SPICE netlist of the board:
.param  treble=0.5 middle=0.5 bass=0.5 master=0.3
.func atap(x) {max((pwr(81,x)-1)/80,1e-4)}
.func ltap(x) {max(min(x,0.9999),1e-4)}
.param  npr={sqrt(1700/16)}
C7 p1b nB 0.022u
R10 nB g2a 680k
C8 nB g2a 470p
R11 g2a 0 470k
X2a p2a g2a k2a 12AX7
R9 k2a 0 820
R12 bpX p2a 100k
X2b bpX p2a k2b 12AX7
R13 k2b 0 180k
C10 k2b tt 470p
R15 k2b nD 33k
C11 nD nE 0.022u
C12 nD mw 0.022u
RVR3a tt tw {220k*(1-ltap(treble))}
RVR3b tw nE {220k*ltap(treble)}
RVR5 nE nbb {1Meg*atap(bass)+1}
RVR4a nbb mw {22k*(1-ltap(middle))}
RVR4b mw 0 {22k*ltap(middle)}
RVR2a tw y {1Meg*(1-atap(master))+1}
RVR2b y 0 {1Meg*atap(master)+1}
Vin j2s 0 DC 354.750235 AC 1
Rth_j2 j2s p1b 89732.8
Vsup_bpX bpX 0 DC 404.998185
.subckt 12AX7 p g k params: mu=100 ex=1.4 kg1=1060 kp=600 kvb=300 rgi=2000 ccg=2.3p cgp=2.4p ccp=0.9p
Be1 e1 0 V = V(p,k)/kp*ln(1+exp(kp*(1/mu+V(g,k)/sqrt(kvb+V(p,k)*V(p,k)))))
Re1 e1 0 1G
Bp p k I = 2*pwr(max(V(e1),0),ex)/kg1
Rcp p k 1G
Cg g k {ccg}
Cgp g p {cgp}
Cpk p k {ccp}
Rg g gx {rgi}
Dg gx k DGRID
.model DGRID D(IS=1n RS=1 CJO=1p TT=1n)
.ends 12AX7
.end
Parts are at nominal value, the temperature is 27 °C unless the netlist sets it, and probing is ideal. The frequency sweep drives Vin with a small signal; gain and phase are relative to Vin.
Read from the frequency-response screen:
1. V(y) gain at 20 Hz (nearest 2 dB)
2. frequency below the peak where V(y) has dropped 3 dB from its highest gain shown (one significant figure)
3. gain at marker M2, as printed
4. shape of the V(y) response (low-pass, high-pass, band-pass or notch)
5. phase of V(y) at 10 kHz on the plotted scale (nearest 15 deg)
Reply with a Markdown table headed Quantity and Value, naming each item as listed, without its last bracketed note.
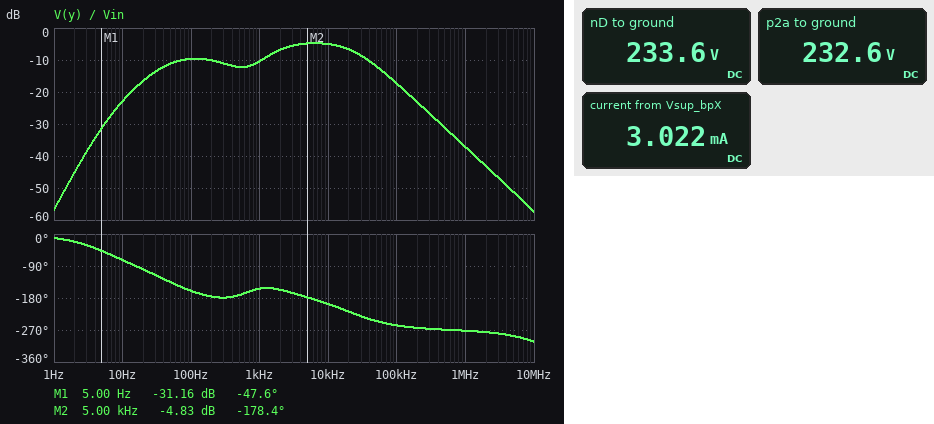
| Quantity | Value |
|---|---|
| V(y) gain at 20 Hz | -16 dB |
| frequency below the peak where V(y) has dropped 3 dB from its highest gain shown | 2 kHz |
| gain at marker M2, as printed | -4.83 dB |
| shape of the V(y) response | band-pass |
| phase of V(y) at 10 kHz on the plotted scale | -195 deg |
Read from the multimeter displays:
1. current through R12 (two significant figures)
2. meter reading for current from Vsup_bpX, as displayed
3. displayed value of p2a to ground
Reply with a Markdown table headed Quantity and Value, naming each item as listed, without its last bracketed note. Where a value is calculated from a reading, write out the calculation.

| Quantity | Value |
|---|---|
| current through R12 | (405 V - 232.6 V) / 100 kΩ = 1.7 mA |
| meter reading for current from Vsup_bpX, as displayed | 3.022 mA |
| displayed value of p2a to ground | 232.6 V |
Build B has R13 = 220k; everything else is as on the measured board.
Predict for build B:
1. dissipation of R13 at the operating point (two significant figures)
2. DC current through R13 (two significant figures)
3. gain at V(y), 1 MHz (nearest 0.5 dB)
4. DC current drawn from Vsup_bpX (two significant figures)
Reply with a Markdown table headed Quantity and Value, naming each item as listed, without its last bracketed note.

| Quantity | Value |
|---|---|
| dissipation of R13 at the operating point | 250 mW |
| DC current through R13 | 1.1 mA |
| gain at V(y), 1 MHz | -37.0 dB |
| DC current drawn from Vsup_bpX | 2.8 mA |
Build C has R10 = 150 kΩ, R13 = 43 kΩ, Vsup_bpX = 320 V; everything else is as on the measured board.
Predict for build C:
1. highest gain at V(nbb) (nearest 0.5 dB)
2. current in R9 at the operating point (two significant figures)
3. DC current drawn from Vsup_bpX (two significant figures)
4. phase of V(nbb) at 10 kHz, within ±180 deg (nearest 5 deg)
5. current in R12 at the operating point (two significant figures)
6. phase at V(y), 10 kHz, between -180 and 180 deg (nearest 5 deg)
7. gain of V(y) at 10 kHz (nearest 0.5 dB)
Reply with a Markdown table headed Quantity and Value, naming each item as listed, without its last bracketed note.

| Quantity | Value |
|---|---|
| highest gain at V(nbb) | 15.0 dB |
| current in R9 at the operating point | 1.3 mA |
| DC current drawn from Vsup_bpX | 5.6 mA |
| phase of V(nbb) at 10 kHz, within ±180 deg | 165 deg |
| current in R12 at the operating point | 1.4 mA |
| phase at V(y), 10 kHz, between -180 and 180 deg | 170 deg |
| gain of V(y) at 10 kHz | -8.0 dB |
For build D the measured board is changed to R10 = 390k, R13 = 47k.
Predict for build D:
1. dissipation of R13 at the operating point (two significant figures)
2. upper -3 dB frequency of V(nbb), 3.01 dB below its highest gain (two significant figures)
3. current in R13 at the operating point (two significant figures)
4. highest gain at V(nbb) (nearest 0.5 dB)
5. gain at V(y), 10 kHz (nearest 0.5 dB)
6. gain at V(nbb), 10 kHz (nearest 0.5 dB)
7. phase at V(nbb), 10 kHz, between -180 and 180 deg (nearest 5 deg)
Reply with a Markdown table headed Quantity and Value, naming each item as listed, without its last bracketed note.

| Quantity | Value |
|---|---|
| dissipation of R13 at the operating point | 1.1 W |
| upper -3 dB frequency of V(nbb), 3.01 dB below its highest gain | 29 kHz |
| current in R13 at the operating point | 4.9 mA |
| highest gain at V(nbb) | 16.5 dB |
| gain at V(y), 10 kHz | -6.5 dB |
| gain at V(nbb), 10 kHz | 16.0 dB |
| phase at V(nbb), 10 kHz, between -180 and 180 deg | 165 deg |
